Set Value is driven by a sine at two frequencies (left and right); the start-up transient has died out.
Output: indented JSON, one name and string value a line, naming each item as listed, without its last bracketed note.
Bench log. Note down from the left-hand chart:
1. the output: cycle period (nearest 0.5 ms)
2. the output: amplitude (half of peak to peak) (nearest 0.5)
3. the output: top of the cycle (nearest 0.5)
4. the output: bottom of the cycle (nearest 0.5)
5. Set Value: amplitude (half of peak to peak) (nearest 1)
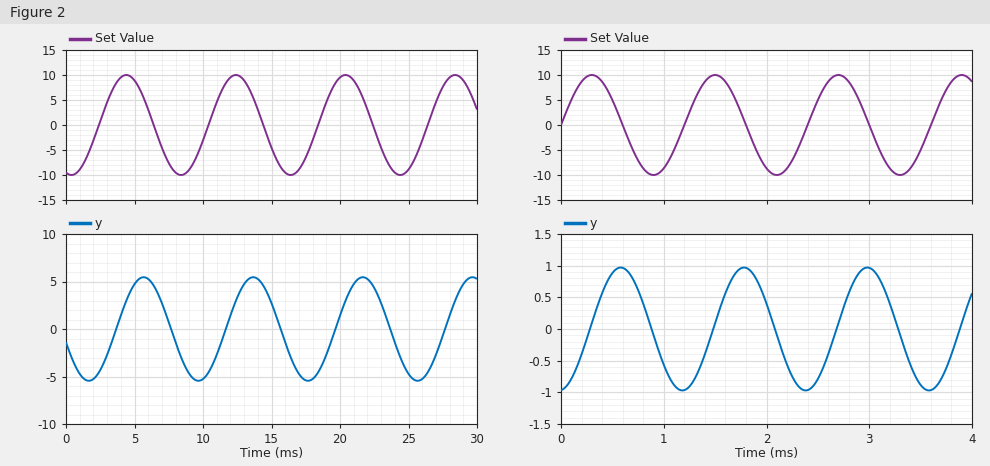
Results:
{
  "the output: cycle period": "8.0 ms",
  "the output: amplitude (half of peak to peak)": "5.5",
  "the output: top of the cycle": "5.5",
  "the output: bottom of the cycle": "-5.5",
  "Set Value: amplitude (half of peak to peak)": "10"
}
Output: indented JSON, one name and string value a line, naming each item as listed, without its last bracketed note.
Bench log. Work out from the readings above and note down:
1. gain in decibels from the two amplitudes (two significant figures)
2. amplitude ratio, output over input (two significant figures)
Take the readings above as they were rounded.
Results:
{
  "gain in decibels from the two amplitudes": "-5.2 dB",
  "amplitude ratio, output over input": "0.55"
}
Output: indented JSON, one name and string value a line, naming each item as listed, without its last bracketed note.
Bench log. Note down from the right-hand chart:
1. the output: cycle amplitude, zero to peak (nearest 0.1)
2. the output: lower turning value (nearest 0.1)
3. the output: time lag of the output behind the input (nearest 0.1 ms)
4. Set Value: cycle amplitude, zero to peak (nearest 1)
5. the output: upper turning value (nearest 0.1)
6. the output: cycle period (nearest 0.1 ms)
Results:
{
  "the output: cycle amplitude, zero to peak": "1.0",
  "the output: lower turning value": "-1.0",
  "the output: time lag of the output behind the input": "0.3 ms",
  "Set Value: cycle amplitude, zero to peak": "10",
  "the output: upper turning value": "1.0",
  "the output: cycle period": "1.2 ms"
}
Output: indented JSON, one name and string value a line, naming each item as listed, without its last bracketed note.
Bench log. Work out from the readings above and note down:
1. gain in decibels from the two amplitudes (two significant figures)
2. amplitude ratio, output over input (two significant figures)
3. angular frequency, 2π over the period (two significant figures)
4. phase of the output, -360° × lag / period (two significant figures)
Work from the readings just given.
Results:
{
  "gain in decibels from the two amplitudes": "-20 dB",
  "amplitude ratio, output over input": "0.10",
  "angular frequency, 2π over the period": "5.2 rad/ms",
  "phase of the output, -360° × lag / period": "-90°"
}
